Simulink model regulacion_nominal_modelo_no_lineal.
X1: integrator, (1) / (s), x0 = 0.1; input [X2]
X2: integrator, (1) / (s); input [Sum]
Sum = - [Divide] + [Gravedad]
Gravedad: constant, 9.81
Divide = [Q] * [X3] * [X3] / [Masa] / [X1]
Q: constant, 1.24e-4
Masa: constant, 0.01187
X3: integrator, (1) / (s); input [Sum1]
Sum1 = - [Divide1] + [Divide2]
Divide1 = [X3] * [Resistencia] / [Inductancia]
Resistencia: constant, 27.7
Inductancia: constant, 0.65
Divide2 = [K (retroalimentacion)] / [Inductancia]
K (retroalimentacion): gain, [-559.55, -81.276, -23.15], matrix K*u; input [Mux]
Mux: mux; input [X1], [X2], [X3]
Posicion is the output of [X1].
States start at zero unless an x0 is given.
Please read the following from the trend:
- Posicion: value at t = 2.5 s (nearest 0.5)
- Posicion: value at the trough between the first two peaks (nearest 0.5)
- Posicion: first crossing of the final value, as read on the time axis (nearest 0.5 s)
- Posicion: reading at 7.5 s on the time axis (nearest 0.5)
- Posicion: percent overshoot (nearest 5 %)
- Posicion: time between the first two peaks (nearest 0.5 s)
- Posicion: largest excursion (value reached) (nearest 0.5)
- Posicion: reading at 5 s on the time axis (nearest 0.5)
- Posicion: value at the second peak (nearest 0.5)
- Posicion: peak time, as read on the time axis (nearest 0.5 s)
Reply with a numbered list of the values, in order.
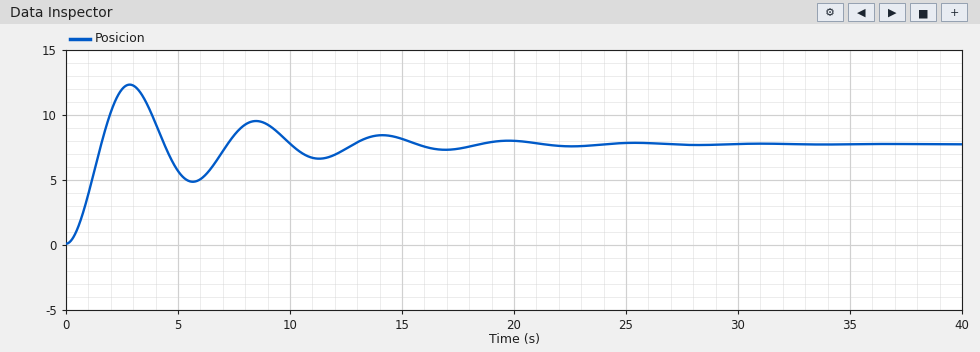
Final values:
1. 12.0
2. 5.0
3. 1.5 s
4. 8.5
5. 60 %
6. 5.5 s
7. 12.5
8. 5.5
9. 9.5
10. 3.0 s
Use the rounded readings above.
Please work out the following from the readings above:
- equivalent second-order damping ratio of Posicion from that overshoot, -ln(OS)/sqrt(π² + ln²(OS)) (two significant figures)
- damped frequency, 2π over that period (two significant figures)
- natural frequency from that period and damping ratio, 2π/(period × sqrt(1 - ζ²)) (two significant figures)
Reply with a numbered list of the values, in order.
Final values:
1. 0.16
2. 1.1 rad/s
3. 1.2 rad/s
